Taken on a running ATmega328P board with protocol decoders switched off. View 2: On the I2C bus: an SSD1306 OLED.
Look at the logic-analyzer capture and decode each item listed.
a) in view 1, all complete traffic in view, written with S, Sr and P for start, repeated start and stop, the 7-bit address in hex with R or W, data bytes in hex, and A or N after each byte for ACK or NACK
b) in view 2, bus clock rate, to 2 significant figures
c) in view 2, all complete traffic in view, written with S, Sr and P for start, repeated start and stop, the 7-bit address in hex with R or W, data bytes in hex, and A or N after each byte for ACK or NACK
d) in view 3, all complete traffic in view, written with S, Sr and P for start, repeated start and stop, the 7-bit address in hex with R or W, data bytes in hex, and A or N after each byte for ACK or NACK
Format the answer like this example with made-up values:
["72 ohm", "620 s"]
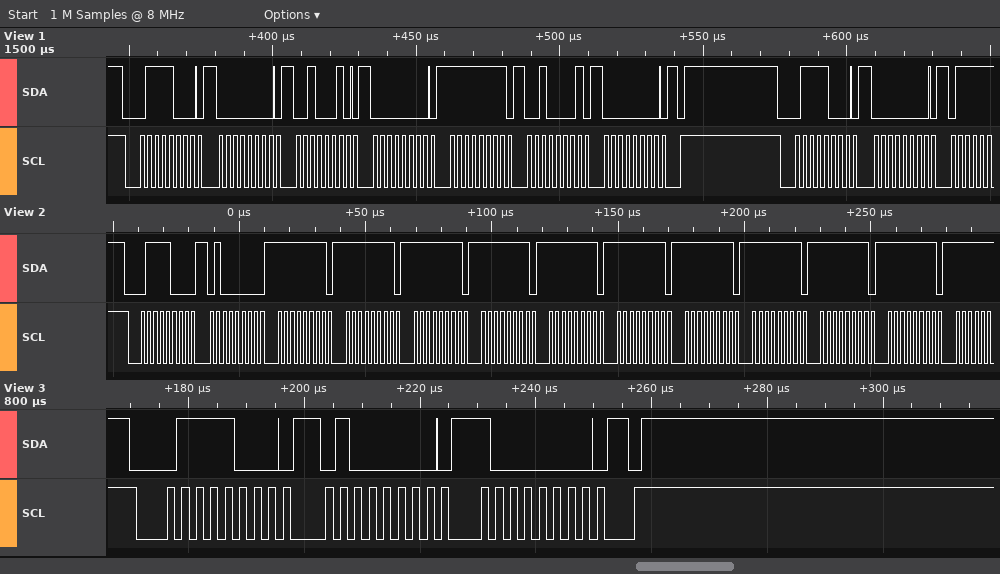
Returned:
["S 3CW A 00 A 22 A 00 A FF A 21 A 00 A P S 3CW A 00 A", "400 kHz", "S 3CW A 40 A FF A FF A FF A FF A FF A FF A FF A FF A FF A FF A", "S 3CW A 40 A 80 A P"]
